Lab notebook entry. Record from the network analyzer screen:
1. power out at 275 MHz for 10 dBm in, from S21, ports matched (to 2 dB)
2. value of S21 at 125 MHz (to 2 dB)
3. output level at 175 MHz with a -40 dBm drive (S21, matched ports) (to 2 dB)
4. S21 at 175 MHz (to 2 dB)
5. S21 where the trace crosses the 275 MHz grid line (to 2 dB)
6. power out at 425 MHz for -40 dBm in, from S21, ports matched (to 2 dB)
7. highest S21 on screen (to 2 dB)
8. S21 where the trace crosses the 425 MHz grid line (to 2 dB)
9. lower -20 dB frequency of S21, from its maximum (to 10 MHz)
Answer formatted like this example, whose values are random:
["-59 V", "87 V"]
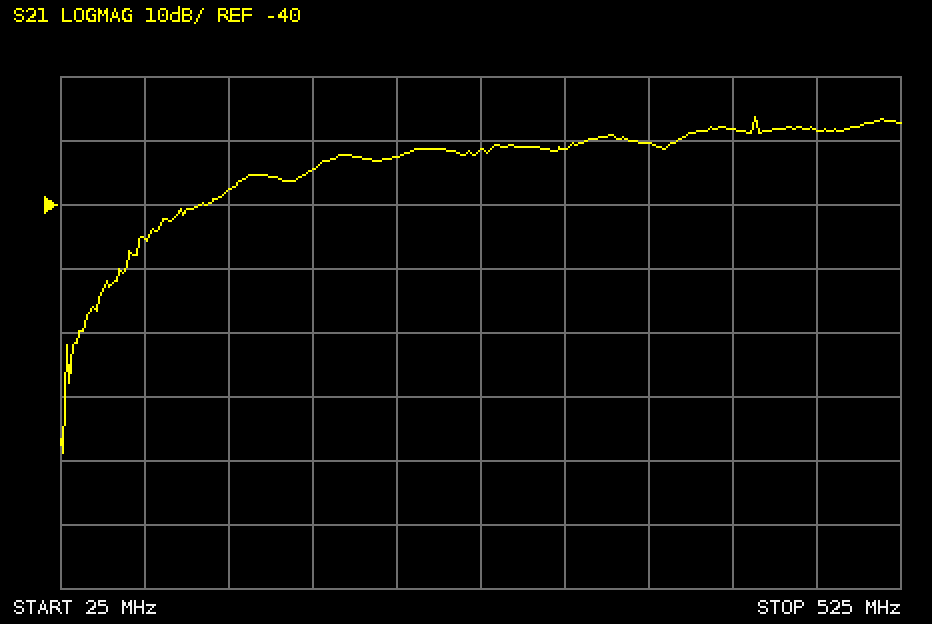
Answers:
["-22 dBm", "-38 dB", "-74 dBm", "-34 dB", "-32 dB", "-68 dBm", "-26 dB", "-28 dB", "70 MHz"]
